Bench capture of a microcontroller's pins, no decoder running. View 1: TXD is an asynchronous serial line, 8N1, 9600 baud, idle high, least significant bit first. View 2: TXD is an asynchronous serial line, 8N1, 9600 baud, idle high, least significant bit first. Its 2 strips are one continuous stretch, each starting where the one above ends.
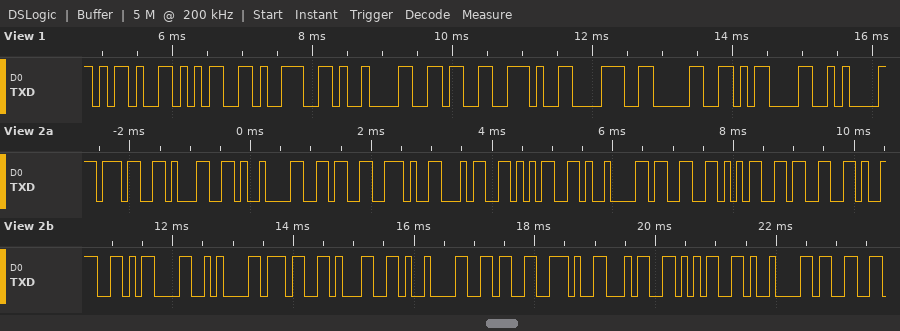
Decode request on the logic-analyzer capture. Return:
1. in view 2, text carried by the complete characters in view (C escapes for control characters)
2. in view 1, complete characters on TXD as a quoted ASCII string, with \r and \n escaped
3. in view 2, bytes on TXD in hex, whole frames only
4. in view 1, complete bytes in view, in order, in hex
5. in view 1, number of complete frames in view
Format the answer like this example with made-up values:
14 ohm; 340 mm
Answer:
"71\t6.45\t3539\r\n71\t6.45\t3"; "-59\t6.80\r\n"; 37 31 09 36 2E 34 35 09 33 35 33 39 0D 0A 37 31 09 36 2E 34 35 09 33; 2D 35 39 09 36 2E 38 30 0D 0A; 10
